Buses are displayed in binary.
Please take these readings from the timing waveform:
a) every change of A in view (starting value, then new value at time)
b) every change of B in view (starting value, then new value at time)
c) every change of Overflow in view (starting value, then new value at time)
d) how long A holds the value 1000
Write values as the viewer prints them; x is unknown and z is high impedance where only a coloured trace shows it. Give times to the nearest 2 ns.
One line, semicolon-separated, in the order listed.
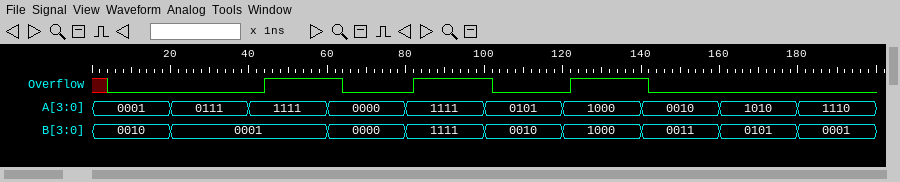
0001, 0111 at 20 ns, 1111 at 40 ns, 0000 at 60 ns, 1111 at 80 ns, 0101 at 100 ns, 1000 at 120 ns, 0010 at 140 ns, 1010 at 160 ns, 1110 at 180 ns; 0010, 0001 at 20 ns, 0000 at 60 ns, 1111 at 80 ns, 0010 at 100 ns, 1000 at 120 ns, 0011 at 140 ns, 0101 at 160 ns, 0001 at 180 ns; x, 0 at 4 ns, 1 at 44 ns, 0 at 64 ns, 1 at 82 ns, 0 at 102 ns, 1 at 122 ns, 0 at 142 ns; 20 ns
